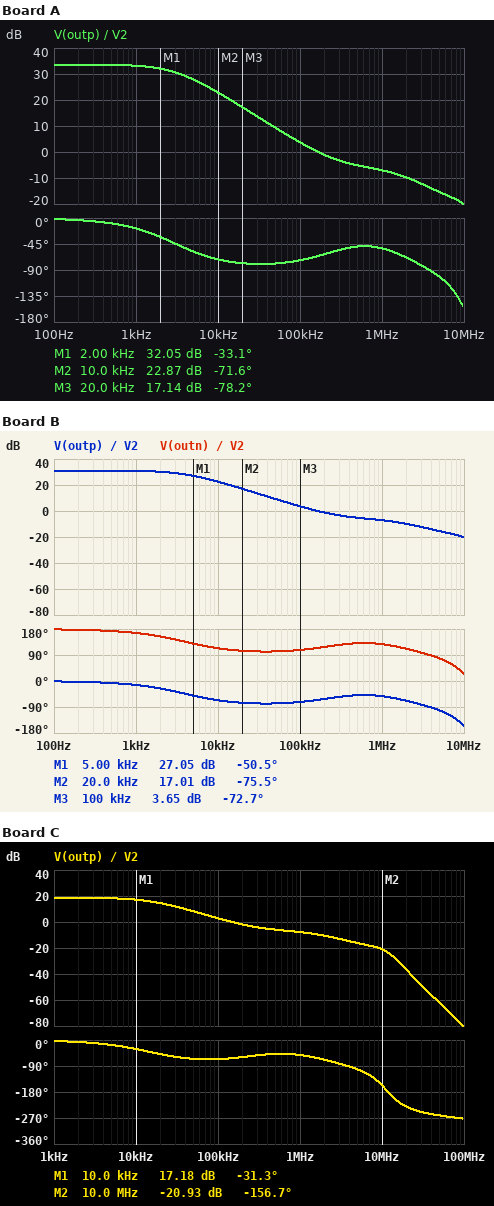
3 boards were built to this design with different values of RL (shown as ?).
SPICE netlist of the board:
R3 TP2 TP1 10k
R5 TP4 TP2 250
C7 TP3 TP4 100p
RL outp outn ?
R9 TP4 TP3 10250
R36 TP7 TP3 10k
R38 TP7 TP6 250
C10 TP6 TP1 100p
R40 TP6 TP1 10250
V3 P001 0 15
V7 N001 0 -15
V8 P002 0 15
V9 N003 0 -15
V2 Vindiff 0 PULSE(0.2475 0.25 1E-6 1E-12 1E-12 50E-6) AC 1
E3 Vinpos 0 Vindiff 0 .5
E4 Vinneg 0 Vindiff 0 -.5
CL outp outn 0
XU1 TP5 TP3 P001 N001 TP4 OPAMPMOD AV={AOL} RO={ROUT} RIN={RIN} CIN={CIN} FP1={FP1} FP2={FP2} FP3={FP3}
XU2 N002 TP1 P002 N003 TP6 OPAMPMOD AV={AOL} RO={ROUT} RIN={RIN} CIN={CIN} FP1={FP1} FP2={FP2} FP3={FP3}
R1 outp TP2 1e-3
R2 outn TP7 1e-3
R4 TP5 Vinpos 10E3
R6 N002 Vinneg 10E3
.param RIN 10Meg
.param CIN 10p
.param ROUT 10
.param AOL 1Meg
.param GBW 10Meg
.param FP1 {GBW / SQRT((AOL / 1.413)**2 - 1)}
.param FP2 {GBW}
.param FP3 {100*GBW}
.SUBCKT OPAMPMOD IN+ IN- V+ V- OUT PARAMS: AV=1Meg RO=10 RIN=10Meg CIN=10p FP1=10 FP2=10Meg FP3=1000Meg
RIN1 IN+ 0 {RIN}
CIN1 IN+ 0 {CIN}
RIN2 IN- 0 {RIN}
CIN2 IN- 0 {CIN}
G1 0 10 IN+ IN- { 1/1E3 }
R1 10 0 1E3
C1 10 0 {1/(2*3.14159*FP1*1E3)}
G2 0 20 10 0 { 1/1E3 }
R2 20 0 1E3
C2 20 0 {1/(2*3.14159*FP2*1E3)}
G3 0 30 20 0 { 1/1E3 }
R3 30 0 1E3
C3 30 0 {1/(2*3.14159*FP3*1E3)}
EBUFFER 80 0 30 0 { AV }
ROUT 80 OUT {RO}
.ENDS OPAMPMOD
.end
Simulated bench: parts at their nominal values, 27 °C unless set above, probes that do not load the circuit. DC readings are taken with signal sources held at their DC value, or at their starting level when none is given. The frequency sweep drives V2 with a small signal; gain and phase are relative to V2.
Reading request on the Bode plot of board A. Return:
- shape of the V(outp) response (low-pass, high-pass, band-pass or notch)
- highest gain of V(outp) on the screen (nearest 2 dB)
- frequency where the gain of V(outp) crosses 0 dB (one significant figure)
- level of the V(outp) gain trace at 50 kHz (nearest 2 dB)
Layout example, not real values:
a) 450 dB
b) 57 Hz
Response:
a) low-pass
b) 34 dB
c) 200 kHz
d) 10 dB
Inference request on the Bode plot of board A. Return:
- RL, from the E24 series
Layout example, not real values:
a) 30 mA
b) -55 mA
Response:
a) 24 kΩ
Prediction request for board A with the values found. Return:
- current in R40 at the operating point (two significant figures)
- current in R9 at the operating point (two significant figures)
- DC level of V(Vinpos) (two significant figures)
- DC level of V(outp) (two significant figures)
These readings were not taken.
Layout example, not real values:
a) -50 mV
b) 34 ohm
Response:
a) 1.2 mA
b) 1.2 mA
c) 120 mV
d) 12 V
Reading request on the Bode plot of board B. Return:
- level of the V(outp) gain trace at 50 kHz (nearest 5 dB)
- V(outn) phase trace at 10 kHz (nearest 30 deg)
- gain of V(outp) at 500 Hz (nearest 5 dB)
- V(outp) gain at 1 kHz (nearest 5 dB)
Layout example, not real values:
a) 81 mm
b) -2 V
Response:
a) 10 dB
b) 120 deg
c) 30 dB
d) 30 dB
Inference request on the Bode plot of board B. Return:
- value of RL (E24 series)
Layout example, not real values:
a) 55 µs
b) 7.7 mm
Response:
a) 18 kΩ
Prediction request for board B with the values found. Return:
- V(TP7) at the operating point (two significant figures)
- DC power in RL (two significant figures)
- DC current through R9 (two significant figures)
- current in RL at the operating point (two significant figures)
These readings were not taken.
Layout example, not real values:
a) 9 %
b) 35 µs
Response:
a) -8.9 V
b) 18 mW
c) 900 µA
d) 990 µA
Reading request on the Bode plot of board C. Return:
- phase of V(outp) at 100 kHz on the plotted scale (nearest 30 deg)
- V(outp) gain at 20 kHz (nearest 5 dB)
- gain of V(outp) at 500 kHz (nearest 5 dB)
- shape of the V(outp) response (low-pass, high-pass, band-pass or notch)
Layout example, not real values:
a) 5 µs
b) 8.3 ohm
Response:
a) -60 deg
b) 15 dB
c) -5 dB
d) low-pass
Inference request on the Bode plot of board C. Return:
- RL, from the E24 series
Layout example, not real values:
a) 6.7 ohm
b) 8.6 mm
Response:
a) 4.3 kΩ
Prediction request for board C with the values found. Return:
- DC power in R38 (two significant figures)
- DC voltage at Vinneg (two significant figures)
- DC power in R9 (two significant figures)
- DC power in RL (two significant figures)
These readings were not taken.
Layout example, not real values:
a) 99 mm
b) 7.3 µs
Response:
a) 370 µW
b) -120 mV
c) 520 µW
d) 4.2 mW
